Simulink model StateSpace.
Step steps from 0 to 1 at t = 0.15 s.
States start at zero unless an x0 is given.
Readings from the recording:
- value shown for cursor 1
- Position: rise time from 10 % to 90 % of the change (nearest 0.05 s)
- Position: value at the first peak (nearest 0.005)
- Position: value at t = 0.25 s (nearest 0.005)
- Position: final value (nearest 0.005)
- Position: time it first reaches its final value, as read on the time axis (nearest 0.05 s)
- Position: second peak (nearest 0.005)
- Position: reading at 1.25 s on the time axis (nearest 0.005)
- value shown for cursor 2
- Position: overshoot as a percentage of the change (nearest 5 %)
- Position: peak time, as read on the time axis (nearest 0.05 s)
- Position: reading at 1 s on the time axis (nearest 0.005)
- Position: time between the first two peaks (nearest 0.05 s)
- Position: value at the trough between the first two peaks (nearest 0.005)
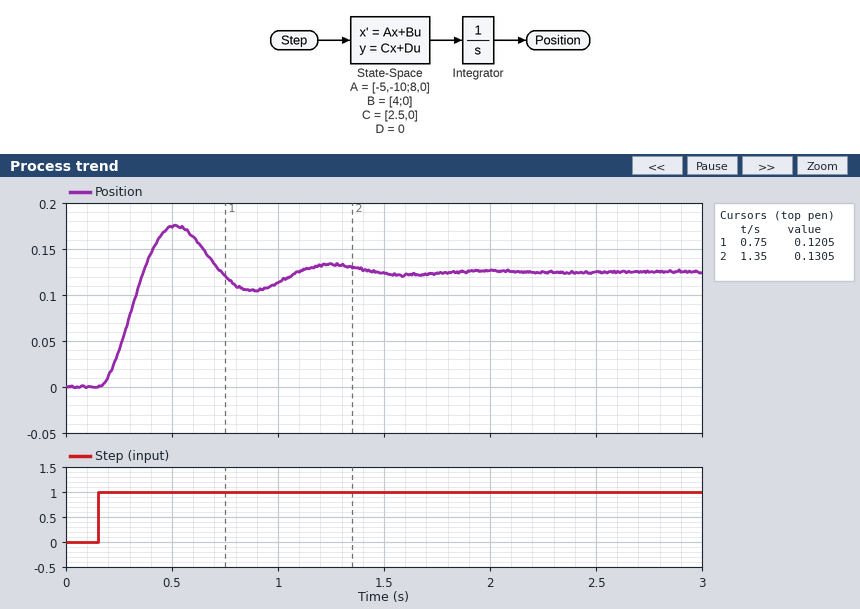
0.1205
0.15 s
0.175
0.040
0.125
0.35 s
0.135
0.135
0.1305
40 %
0.50 s
0.115
0.75 s
0.105
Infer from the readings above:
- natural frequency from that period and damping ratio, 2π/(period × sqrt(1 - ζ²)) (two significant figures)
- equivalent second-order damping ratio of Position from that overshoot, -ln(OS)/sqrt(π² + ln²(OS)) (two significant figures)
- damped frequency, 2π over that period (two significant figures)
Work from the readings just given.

8.7 rad/s
0.28
8.4 rad/s
